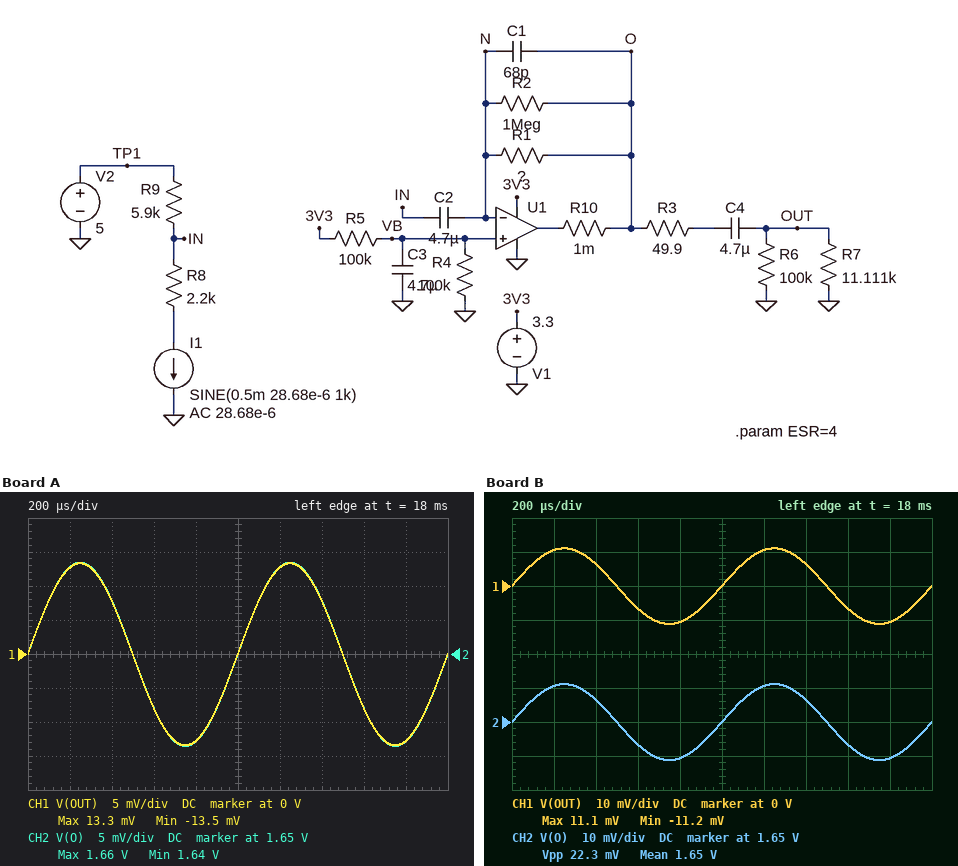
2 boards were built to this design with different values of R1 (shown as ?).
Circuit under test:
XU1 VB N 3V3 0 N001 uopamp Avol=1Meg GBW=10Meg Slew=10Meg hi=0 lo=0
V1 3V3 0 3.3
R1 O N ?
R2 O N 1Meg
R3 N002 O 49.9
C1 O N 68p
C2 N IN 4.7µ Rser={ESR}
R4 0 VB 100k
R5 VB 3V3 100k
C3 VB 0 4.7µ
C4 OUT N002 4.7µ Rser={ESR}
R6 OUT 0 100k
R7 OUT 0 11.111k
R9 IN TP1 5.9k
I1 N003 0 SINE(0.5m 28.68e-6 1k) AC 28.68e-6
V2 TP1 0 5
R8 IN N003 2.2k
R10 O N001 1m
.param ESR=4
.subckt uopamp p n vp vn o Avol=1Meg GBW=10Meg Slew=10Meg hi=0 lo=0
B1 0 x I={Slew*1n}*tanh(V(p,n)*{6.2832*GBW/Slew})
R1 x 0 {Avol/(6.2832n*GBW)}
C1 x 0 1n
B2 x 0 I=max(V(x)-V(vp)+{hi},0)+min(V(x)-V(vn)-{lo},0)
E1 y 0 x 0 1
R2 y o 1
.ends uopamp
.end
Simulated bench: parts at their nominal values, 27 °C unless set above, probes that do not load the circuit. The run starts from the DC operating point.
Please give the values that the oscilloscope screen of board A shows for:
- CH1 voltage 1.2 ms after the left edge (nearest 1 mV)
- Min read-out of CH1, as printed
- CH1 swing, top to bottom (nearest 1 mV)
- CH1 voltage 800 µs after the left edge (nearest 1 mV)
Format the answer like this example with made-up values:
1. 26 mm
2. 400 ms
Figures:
1. 13 mV
2. -13.5 mV
3. 27 mV
4. -13 mV
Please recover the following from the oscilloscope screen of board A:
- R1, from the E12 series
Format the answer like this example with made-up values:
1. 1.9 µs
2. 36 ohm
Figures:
1. 470 Ω
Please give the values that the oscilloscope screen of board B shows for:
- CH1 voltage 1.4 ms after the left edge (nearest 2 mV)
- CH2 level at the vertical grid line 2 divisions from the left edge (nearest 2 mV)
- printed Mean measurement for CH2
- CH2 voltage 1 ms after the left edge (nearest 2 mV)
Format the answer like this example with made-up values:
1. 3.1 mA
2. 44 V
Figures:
1. 6 mV
2. 1.656 V
3. 1.65 V
4. 1.650 V
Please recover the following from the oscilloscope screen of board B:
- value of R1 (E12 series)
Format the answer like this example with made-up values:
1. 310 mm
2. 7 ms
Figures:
1. 390 Ω
